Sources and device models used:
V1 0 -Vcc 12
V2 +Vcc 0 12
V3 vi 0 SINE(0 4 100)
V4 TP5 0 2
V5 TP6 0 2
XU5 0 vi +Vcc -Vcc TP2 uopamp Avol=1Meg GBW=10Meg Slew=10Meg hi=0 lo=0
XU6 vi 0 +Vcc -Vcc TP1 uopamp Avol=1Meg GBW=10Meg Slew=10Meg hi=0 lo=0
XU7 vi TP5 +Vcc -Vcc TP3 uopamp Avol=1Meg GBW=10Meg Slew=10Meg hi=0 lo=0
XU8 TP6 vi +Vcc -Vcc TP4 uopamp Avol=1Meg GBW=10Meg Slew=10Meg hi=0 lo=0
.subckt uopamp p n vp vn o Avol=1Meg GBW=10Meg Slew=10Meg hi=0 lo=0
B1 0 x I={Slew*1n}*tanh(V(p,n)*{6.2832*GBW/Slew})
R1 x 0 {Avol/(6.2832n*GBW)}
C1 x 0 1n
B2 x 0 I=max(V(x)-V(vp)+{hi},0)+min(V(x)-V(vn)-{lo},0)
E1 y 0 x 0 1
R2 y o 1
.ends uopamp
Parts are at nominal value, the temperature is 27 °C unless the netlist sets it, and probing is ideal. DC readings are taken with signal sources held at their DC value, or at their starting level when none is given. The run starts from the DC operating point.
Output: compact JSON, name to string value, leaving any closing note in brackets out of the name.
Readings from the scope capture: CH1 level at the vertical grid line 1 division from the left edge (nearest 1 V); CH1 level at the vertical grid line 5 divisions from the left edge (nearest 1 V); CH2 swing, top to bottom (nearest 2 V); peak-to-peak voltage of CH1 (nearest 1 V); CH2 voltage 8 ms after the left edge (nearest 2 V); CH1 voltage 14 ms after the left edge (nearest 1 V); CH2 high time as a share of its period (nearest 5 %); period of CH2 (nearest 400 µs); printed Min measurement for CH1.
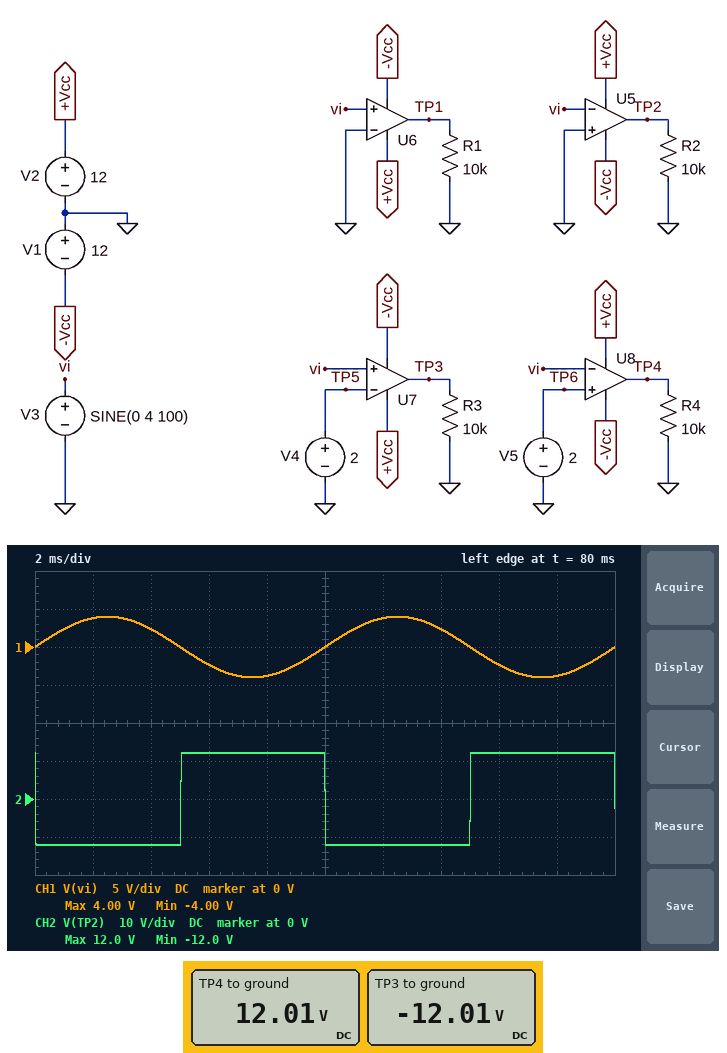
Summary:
{"CH1 level at the vertical grid line 1 division from the left edge": "4 V", "CH1 level at the vertical grid line 5 divisions from the left edge": "0 V", "CH2 swing, top to bottom": "24 V", "peak-to-peak voltage of CH1": "8 V", "CH2 voltage 8 ms after the left edge": "12 V", "CH1 voltage 14 ms after the left edge": "2 V", "CH2 high time as a share of its period": "50 %", "period of CH2": "10.0 ms", "printed Min measurement for CH1": "-4.00 V"}
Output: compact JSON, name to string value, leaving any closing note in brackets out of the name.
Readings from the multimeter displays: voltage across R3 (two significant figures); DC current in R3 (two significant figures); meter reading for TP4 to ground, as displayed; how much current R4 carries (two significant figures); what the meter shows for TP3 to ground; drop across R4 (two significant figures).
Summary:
{"voltage across R3": "12 V", "DC current in R3": "1.2 mA", "meter reading for TP4 to ground, as displayed": "12.01 V", "how much current R4 carries": "1.2 mA", "what the meter shows for TP3 to ground": "-12.01 V", "drop across R4": "12 V"}
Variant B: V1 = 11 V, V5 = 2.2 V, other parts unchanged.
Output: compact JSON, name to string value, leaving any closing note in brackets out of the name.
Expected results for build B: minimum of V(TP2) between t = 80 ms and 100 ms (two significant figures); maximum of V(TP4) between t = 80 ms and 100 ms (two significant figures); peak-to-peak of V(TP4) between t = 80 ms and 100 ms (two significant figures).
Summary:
{"minimum of V(TP2) between t = 80 ms and 100 ms": "-11 V", "maximum of V(TP4) between t = 80 ms and 100 ms": "12 V", "peak-to-peak of V(TP4) between t = 80 ms and 100 ms": "23 V"}
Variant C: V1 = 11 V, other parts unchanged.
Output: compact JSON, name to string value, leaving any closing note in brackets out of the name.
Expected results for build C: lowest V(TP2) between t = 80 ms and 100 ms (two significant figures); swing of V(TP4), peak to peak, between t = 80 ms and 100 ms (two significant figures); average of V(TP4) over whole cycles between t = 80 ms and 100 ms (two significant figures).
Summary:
{"lowest V(TP2) between t = 80 ms and 100 ms": "-11 V", "swing of V(TP4), peak to peak, between t = 80 ms and 100 ms": "23 V", "average of V(TP4) over whole cycles between t = 80 ms and 100 ms": "4.3 V"}
